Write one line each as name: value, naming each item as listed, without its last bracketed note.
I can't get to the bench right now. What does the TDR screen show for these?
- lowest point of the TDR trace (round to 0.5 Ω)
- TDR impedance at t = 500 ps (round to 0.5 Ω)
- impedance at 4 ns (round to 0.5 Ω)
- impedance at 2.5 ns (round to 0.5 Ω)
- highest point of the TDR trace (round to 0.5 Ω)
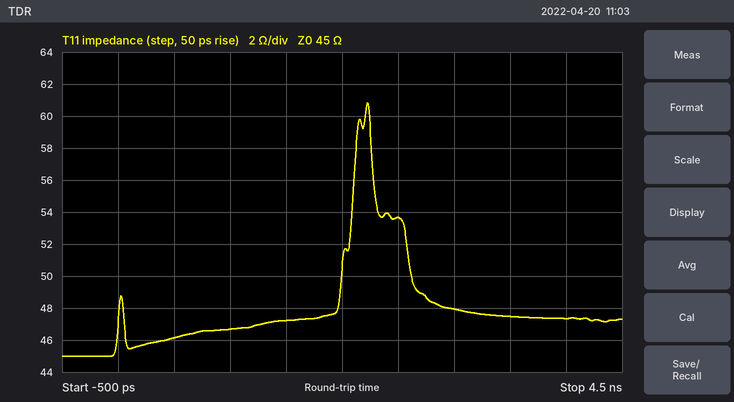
lowest point of the TDR trace: 45.0 Ω
TDR impedance at t = 500 ps: 46.0 Ω
impedance at 4 ns: 47.5 Ω
impedance at 2.5 ns: 53.5 Ω
highest point of the TDR trace: 61.0 Ω
